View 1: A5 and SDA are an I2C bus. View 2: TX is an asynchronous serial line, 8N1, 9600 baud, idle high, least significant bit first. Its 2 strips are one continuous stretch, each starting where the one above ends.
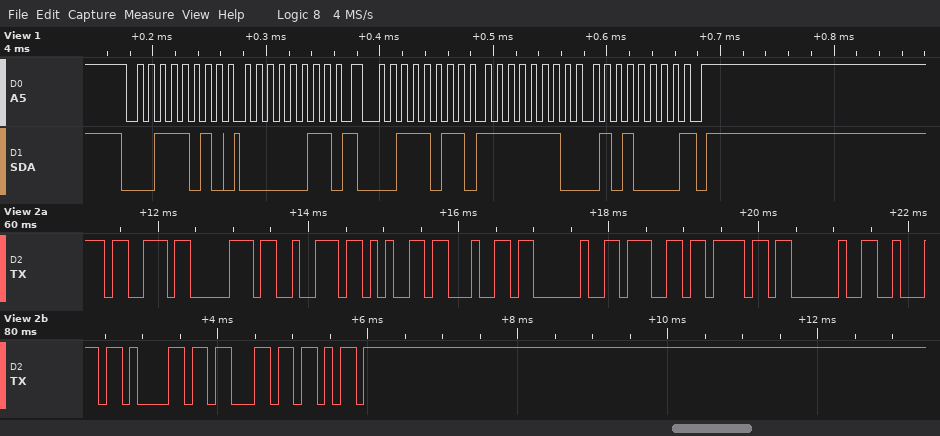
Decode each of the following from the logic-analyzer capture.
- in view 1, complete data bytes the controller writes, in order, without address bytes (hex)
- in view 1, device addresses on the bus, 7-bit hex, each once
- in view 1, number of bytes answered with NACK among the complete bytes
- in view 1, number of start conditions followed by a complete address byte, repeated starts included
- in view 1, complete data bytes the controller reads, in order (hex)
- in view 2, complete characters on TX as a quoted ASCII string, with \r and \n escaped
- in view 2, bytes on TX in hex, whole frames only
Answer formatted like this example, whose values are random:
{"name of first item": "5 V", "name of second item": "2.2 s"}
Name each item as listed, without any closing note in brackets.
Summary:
{"in view 1, complete data bytes the controller writes, in order, without address bytes": "03", "in view 1, device addresses on the bus, 7-bit hex, each once": "0x1D", "in view 1, number of bytes answered with NACK among the complete bytes": "1", "in view 1, number of start conditions followed by a complete address byte, repeated starts included": "2", "in view 1, complete data bytes the controller reads, in order": "FE 50", "in view 2, complete characters on TX as a quoted ASCII string, with \\r and \\n escaped": "\"spred go back\"", "in view 2, bytes on TX in hex, whole frames only": "73 70 72 65 64 20 67 6F 20 62 61 63 6B"}
